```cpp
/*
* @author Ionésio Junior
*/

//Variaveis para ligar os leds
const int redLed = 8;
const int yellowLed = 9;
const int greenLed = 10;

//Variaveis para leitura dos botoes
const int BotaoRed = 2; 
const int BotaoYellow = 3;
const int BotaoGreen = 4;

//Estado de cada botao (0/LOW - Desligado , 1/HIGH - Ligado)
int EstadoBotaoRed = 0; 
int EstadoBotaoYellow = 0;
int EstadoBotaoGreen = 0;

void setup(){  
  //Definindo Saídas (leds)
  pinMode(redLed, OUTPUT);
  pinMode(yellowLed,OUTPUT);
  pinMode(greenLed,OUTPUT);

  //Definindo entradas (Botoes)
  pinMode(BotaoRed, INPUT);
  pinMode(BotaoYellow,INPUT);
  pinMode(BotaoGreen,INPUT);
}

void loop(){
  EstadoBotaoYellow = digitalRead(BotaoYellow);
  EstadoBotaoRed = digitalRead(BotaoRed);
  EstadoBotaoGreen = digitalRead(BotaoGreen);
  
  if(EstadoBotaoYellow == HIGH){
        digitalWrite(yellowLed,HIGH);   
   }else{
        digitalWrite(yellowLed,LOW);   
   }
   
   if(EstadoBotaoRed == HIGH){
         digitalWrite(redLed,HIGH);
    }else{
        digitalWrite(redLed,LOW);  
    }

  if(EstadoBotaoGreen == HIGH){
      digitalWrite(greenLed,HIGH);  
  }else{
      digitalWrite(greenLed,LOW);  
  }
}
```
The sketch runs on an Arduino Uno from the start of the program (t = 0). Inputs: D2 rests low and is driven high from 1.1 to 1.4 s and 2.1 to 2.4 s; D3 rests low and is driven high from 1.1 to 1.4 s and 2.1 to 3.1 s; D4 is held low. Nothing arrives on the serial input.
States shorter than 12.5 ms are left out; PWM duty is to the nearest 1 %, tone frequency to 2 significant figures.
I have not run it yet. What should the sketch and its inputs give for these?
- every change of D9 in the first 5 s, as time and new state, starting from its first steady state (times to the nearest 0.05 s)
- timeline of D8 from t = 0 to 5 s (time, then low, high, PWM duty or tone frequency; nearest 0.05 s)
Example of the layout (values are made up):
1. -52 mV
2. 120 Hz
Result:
1. 0 s low; 1.1 s high; 1.4 s low; 2.1 s high; 3.1 s low
2. 0 s low; 1.1 s high; 1.4 s low; 2.1 s high; 2.4 s low
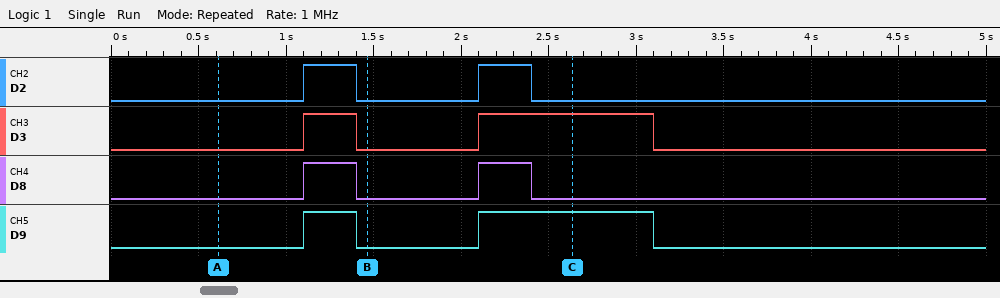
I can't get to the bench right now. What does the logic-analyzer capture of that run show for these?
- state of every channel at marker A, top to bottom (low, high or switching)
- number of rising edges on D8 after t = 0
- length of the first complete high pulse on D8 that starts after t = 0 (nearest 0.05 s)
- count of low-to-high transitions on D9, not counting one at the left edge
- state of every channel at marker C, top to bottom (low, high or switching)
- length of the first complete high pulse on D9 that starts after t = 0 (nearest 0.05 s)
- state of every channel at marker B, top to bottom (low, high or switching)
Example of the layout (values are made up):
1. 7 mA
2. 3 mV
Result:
1. D2 low, D3 low, D8 low, D9 low
2. 2
3. 0.30 s
4. 2
5. D2 low, D3 high, D8 low, D9 high
6. 0.30 s
7. D2 low, D3 low, D8 low, D9 low
